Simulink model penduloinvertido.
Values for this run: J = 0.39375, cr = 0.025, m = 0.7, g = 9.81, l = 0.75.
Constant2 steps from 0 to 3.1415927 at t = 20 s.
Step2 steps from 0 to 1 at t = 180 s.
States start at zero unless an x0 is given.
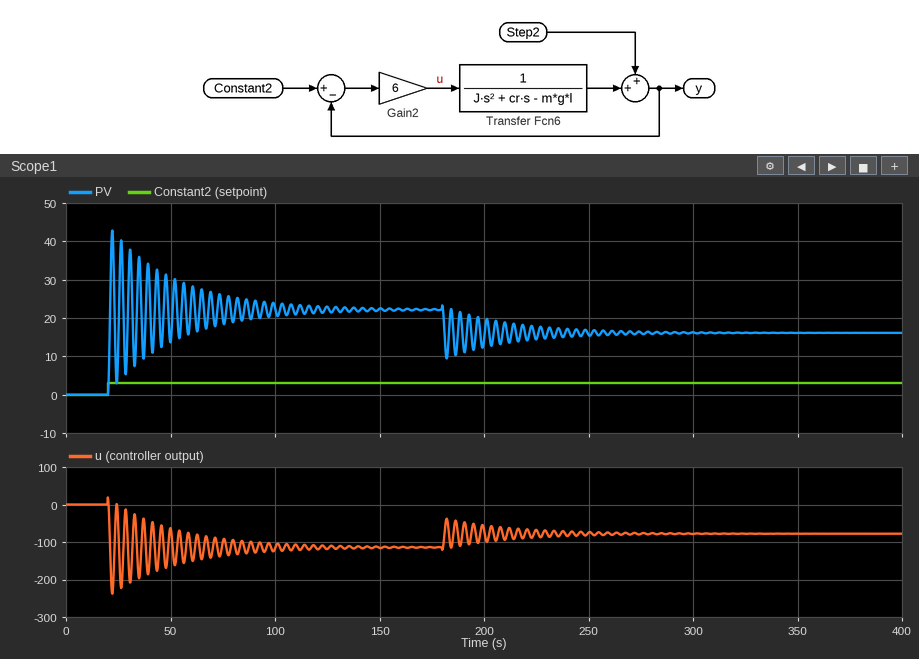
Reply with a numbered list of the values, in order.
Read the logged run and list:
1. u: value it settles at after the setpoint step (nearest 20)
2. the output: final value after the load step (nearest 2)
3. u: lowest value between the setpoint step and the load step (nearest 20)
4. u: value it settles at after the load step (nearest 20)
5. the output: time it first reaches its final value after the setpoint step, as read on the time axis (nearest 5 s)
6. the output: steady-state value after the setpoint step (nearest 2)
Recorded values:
1. -120
2. 16
3. -240
4. -80
5. 20 s
6. 22
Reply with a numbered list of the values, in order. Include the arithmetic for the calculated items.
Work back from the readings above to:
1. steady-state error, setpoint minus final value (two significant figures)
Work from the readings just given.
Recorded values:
1. 3.14159 - 22 = -19
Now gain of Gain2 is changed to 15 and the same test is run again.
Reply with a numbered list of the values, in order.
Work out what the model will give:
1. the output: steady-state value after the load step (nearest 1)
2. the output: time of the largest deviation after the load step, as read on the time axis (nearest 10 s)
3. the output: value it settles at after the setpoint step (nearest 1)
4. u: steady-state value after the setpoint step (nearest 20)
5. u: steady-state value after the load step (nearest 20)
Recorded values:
1. 4
2. 180 s
3. 5
4. -20
5. -20
